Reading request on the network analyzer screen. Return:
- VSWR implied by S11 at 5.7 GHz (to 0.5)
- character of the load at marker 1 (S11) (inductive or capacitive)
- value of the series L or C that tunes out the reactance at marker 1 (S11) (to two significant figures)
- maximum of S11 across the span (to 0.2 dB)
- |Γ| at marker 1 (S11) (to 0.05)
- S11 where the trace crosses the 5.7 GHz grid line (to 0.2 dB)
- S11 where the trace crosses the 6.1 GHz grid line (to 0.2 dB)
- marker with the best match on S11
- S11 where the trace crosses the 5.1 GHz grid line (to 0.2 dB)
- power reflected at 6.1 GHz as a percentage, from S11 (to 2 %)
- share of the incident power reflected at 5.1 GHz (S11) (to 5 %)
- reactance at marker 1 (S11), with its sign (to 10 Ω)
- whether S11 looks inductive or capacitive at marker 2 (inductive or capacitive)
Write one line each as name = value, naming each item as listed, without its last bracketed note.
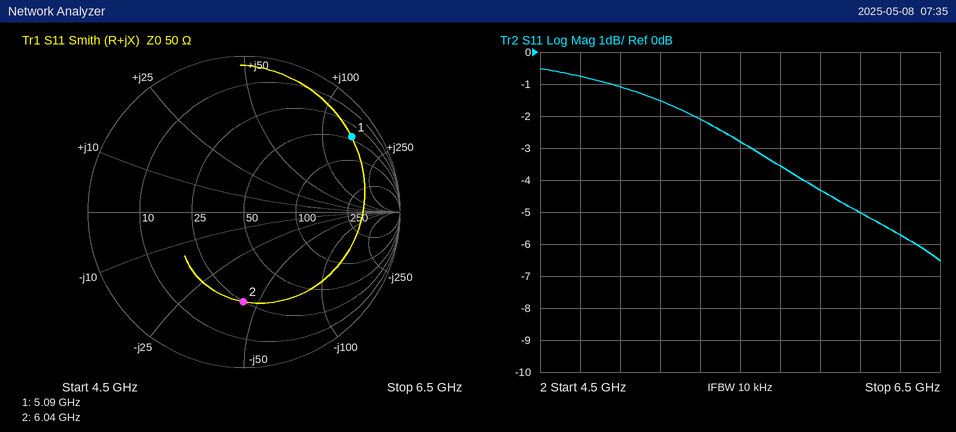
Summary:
VSWR implied by S11 at 5.7 GHz = 5.0
character of the load at marker 1 (S11) = inductive
value of the series L or C that tunes out the reactance at marker 1 (S11) = 210 fF
maximum of S11 across the span = -0.6 dB
|Γ| at marker 1 (S11) = 0.85
S11 where the trace crosses the 5.7 GHz grid line = -3.6 dB
S11 where the trace crosses the 6.1 GHz grid line = -5.0 dB
marker with the best match on S11 = marker 2
S11 where the trace crosses the 5.1 GHz grid line = -1.6 dB
power reflected at 6.1 GHz as a percentage, from S11 = 32 %
share of the incident power reflected at 5.1 GHz (S11) = 70 %
reactance at marker 1 (S11), with its sign = +150 Ω
whether S11 looks inductive or capacitive at marker 2 = capacitive
